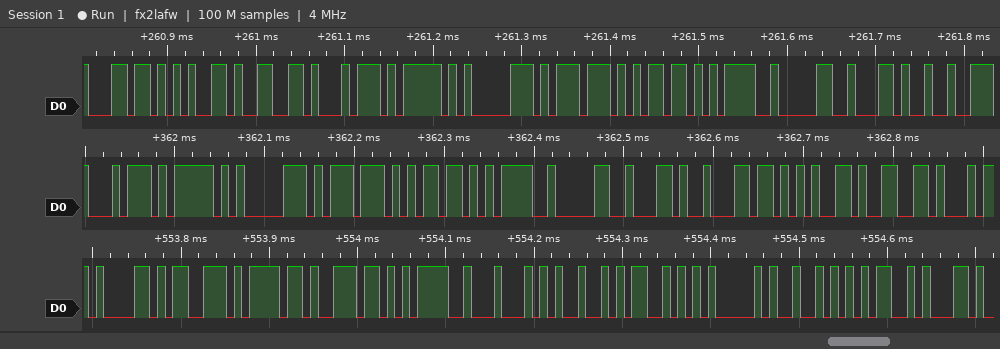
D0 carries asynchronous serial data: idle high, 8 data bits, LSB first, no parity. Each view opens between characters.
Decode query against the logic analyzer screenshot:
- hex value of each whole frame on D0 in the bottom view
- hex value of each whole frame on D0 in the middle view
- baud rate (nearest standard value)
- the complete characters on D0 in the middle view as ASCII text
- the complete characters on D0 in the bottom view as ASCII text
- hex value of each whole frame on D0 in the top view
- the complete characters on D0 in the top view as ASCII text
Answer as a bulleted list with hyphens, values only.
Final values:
- 61, 73, 6F, 6E, 3D, 44, 49, 53, 41, 52, 4D
- 74, 5F, 70, 77, 6D, 3D, 30, 2C, 6C, 65, 66
- 115200 baud
- "t_pwm=0,lef"
- "ason=DISARM"
- 6C, 65, 66, 74, 5F, 70, 77, 6D, 3D, 30, 2C
- "left_pwm=0,"
